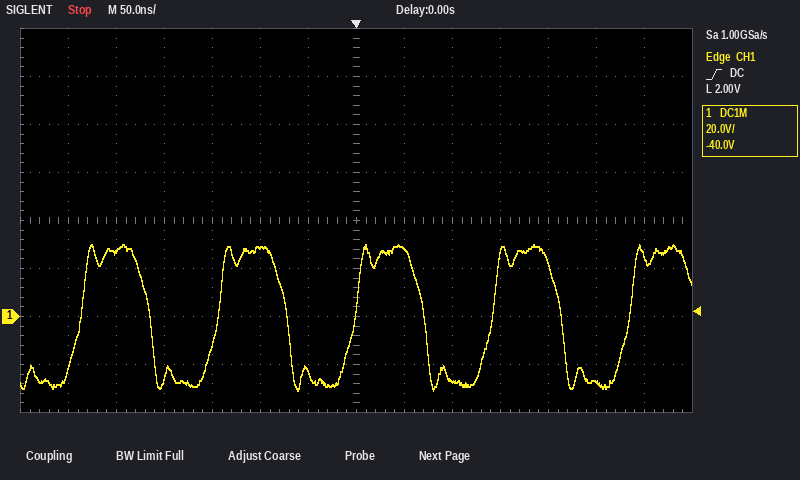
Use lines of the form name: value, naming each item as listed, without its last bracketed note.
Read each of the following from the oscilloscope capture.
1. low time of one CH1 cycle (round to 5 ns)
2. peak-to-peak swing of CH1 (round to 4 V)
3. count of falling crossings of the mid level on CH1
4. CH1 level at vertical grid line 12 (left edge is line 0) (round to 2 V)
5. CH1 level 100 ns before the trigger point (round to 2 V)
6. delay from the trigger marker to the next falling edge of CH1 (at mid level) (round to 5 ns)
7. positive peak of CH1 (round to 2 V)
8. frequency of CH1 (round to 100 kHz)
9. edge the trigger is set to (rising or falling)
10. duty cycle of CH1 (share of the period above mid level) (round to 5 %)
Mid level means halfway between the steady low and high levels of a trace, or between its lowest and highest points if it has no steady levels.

low time of one CH1 cycle: 70 ns
peak-to-peak swing of CH1: 60 V
count of falling crossings of the mid level on CH1: 4
CH1 level at vertical grid line 12 (left edge is line 0): -28 V
CH1 level 100 ns before the trigger point: 28 V
delay from the trigger marker to the next falling edge of CH1 (at mid level): 70 ns
positive peak of CH1: 30 V
frequency of CH1: 7.0 MHz
edge the trigger is set to: rising
duty cycle of CH1 (share of the period above mid level): 50 %
